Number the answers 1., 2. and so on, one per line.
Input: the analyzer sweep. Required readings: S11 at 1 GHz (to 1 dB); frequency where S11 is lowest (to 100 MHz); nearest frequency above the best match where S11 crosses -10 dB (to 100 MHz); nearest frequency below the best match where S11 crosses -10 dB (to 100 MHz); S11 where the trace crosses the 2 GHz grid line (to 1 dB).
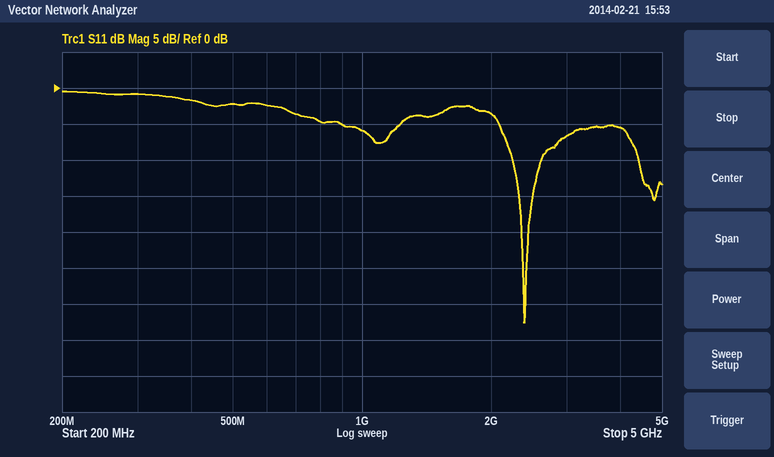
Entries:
1. -6 dB
2. 2.4 GHz
3. 2.6 GHz
4. 2.2 GHz
5. -4 dB
